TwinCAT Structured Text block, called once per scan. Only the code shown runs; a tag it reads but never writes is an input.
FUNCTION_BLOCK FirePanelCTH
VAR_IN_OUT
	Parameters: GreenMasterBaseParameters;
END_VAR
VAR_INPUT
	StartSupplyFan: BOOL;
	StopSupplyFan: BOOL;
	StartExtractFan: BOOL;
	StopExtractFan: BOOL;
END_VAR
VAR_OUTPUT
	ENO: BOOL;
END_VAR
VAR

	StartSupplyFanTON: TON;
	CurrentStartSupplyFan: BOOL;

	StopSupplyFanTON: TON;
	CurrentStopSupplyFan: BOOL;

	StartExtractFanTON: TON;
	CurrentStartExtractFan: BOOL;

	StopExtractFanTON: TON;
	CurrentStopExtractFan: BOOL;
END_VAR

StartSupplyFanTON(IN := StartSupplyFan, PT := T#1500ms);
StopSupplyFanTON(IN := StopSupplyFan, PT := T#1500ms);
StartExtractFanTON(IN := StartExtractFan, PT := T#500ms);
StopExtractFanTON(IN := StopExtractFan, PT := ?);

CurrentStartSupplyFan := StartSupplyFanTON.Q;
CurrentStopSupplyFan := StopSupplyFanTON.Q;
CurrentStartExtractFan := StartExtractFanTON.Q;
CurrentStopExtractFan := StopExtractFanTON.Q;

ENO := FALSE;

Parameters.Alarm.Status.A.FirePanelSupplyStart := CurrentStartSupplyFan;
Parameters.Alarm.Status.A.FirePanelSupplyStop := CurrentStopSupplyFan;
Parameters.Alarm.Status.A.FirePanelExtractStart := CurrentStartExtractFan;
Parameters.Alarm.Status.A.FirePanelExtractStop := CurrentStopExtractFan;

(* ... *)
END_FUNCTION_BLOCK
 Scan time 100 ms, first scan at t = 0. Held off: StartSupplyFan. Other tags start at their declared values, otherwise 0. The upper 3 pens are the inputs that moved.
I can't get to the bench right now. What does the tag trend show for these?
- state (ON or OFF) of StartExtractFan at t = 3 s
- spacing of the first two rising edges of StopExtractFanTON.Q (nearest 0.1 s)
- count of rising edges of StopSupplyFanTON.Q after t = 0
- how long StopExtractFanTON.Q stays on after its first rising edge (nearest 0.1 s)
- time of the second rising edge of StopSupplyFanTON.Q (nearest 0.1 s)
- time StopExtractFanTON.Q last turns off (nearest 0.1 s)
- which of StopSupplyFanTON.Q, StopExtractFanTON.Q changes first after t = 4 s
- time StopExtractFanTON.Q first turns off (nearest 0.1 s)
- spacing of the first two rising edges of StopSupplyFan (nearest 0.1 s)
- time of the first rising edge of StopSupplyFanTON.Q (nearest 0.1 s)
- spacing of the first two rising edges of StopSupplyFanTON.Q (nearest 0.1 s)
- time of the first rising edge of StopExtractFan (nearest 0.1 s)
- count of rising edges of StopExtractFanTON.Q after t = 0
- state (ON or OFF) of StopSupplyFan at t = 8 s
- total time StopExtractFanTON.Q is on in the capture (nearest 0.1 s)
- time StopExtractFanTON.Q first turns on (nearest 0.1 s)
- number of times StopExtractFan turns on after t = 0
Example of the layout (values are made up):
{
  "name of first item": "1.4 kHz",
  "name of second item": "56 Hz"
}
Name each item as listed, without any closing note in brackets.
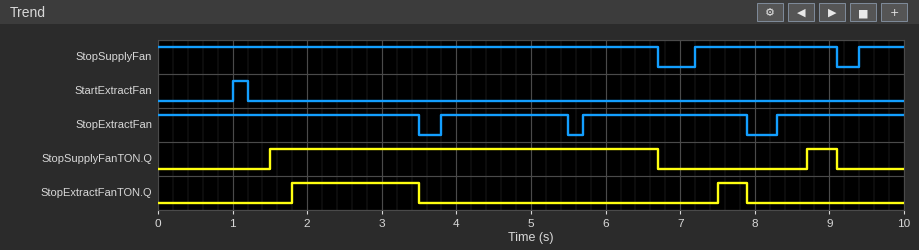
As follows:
{
  "state (ON or OFF) of StartExtractFan at t = 3 s": "OFF",
  "spacing of the first two rising edges of StopExtractFanTON.Q": "5.7 s",
  "count of rising edges of StopSupplyFanTON.Q after t = 0": "2",
  "how long StopExtractFanTON.Q stays on after its first rising edge": "1.7 s",
  "time of the second rising edge of StopSupplyFanTON.Q": "8.7 s",
  "time StopExtractFanTON.Q last turns off": "7.9 s",
  "which of StopSupplyFanTON.Q, StopExtractFanTON.Q changes first after t = 4 s": "StopSupplyFanTON.Q",
  "time StopExtractFanTON.Q first turns off": "3.5 s",
  "spacing of the first two rising edges of StopSupplyFan": "2.2 s",
  "time of the first rising edge of StopSupplyFanTON.Q": "1.5 s",
  "spacing of the first two rising edges of StopSupplyFanTON.Q": "7.2 s",
  "time of the first rising edge of StopExtractFan": "3.8 s",
  "count of rising edges of StopExtractFanTON.Q after t = 0": "2",
  "state (ON or OFF) of StopSupplyFan at t = 8 s": "ON",
  "total time StopExtractFanTON.Q is on in the capture": "2.1 s",
  "time StopExtractFanTON.Q first turns on": "1.8 s",
  "number of times StopExtractFan turns on after t = 0": "3"
}
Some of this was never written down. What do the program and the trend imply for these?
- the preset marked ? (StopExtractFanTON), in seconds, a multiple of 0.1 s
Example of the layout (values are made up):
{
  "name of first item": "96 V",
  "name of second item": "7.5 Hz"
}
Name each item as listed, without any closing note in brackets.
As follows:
{
  "the preset marked ? (StopExtractFanTON), in seconds, a multiple of 0.1 s": "1.8 s"
}
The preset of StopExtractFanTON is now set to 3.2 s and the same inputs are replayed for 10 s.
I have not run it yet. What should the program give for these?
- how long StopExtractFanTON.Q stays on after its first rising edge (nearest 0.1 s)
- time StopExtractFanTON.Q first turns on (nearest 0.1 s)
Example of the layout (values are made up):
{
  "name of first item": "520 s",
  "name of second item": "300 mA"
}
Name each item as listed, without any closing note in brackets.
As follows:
{
  "how long StopExtractFanTON.Q stays on after its first rising edge": "0.3 s",
  "time StopExtractFanTON.Q first turns on": "3.2 s"
}
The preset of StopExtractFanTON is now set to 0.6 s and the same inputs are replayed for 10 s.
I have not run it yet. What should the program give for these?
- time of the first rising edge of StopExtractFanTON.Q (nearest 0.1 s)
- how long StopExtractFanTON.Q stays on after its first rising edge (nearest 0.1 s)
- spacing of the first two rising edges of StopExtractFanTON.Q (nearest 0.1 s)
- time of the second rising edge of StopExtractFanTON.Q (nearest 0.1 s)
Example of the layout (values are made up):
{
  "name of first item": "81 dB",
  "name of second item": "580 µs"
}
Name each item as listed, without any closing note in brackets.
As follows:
{
  "time of the first rising edge of StopExtractFanTON.Q": "0.6 s",
  "how long StopExtractFanTON.Q stays on after its first rising edge": "2.9 s",
  "spacing of the first two rising edges of StopExtractFanTON.Q": "3.8 s",
  "time of the second rising edge of StopExtractFanTON.Q": "4.4 s"
}
